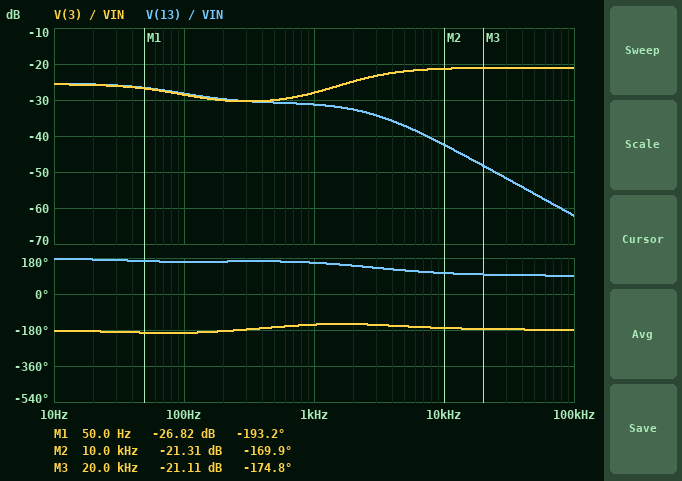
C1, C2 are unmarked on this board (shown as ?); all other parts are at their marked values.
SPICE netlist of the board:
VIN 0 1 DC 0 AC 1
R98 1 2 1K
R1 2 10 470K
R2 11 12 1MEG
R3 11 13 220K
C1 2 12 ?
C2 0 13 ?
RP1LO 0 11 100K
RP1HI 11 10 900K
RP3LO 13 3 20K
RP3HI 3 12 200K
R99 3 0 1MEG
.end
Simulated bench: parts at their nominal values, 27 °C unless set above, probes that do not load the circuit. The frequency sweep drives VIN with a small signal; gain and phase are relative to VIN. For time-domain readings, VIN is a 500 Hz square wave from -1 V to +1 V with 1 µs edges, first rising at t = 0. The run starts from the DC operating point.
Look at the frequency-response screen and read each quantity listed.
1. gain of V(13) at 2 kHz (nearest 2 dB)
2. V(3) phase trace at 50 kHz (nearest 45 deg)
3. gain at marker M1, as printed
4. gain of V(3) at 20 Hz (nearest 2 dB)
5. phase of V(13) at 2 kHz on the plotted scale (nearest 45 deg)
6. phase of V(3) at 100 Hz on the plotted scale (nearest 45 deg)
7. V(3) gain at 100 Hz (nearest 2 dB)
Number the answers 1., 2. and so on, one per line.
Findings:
1. -32 dB
2. -180 deg
3. -26.82 dB
4. -26 dB
5. 135 deg
6. -180 deg
7. -28 dB
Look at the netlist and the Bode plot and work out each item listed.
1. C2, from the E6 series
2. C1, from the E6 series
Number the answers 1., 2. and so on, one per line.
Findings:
1. 10 nF
2. 330 pF
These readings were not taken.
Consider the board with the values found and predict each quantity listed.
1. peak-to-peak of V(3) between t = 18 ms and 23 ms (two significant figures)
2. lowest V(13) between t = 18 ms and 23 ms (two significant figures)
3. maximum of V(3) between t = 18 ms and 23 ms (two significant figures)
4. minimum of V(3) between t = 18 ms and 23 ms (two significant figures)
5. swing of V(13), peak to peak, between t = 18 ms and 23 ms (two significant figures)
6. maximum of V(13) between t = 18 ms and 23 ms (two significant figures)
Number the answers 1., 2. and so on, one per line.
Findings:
1. 290 mV
2. -34 mV
3. 140 mV
4. -140 mV
5. 68 mV
6. 34 mV
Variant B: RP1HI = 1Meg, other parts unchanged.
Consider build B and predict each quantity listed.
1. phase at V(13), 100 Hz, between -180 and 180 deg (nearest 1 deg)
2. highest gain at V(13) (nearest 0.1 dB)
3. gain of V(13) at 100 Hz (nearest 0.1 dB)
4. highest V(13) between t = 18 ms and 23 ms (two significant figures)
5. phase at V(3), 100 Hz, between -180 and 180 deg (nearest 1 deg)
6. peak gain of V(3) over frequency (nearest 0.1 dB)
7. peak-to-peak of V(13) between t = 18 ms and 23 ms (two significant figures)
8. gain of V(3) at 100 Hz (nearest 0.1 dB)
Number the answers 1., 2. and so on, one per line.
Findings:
1. 162 deg
2. -26.0 dB
3. -28.6 dB
4. 33 mV
5. 168 deg
6. -21.0 dB
7. 66 mV
8. -28.9 dB
